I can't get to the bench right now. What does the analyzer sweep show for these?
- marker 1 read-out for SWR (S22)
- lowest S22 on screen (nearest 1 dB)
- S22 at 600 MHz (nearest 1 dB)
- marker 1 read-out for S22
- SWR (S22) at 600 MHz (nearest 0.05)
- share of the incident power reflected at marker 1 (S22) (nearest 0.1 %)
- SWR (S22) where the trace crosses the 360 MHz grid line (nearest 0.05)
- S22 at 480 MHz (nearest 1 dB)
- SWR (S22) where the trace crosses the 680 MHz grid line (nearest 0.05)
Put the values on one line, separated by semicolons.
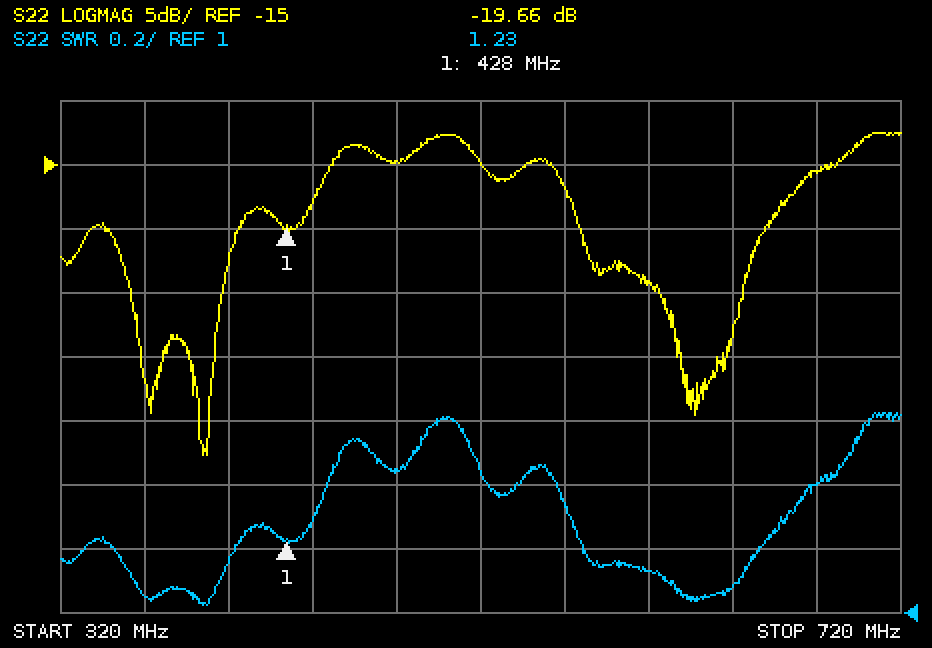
1.23; -38 dB; -24 dB; -19.66 dB; 1.15; 1.1 %; 1.05; -15 dB; 1.40
